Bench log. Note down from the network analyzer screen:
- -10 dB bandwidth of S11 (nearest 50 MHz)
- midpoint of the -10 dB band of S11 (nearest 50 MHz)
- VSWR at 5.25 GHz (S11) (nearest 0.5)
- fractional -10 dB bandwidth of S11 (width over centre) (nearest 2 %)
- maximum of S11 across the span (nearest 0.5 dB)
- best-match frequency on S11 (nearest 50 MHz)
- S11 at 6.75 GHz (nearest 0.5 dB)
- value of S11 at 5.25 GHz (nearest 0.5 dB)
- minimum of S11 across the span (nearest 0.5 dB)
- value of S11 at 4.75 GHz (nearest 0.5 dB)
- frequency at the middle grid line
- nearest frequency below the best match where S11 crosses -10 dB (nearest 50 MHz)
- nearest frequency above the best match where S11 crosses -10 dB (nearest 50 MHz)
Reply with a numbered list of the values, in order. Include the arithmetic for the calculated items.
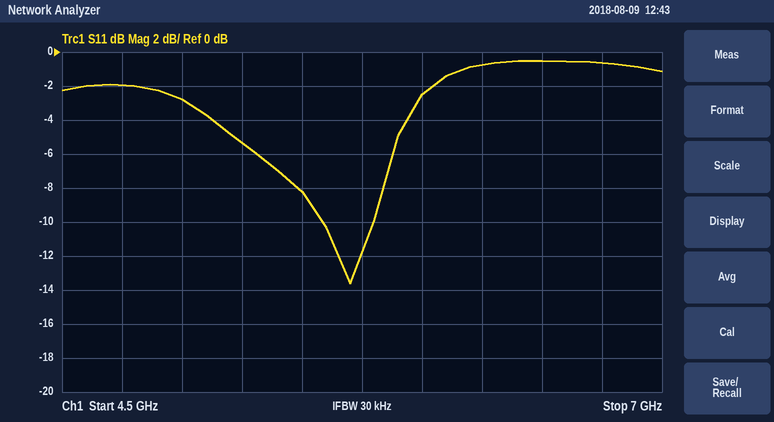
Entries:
1. 5.80 GHz − 5.60 GHz = 200 MHz
2. 5.70 GHz
3. |Γ| = 10^(-5.5/20) = 0.5309; VSWR = (1 + 0.5309)/(1 − 0.5309) ≈ 3.26, so 3.5 to the nearest 0.5
4. 200 MHz / 5.7 GHz ≈ 4 %
5. -0.5 dB
6. 5.70 GHz
7. -0.5 dB
8. -5.5 dB
9. -13.5 dB
10. -2.0 dB
11. 5.75 GHz
12. 5.60 GHz
13. 5.80 GHz
